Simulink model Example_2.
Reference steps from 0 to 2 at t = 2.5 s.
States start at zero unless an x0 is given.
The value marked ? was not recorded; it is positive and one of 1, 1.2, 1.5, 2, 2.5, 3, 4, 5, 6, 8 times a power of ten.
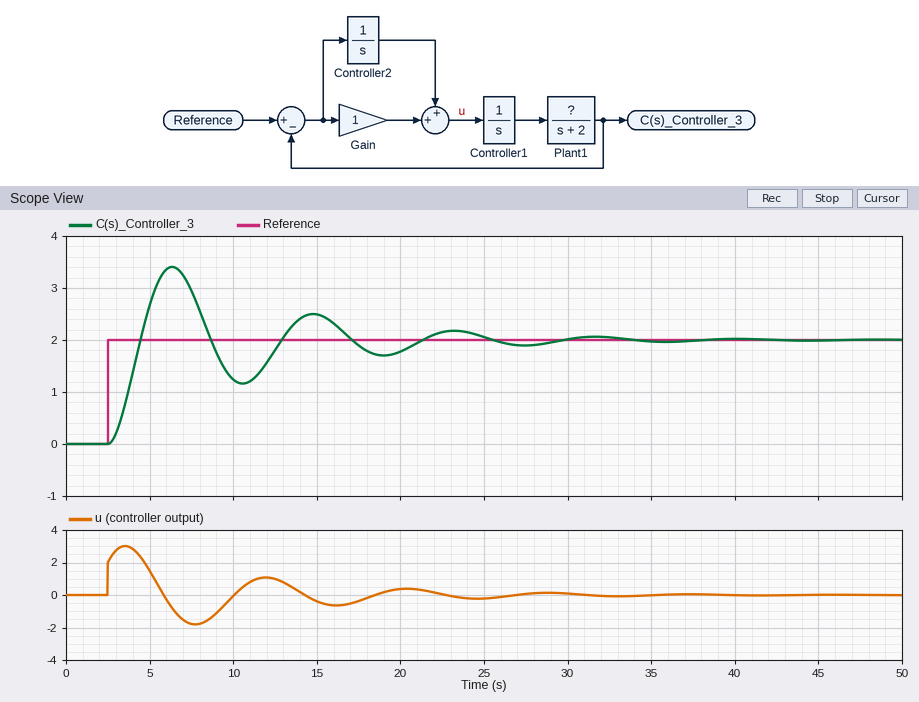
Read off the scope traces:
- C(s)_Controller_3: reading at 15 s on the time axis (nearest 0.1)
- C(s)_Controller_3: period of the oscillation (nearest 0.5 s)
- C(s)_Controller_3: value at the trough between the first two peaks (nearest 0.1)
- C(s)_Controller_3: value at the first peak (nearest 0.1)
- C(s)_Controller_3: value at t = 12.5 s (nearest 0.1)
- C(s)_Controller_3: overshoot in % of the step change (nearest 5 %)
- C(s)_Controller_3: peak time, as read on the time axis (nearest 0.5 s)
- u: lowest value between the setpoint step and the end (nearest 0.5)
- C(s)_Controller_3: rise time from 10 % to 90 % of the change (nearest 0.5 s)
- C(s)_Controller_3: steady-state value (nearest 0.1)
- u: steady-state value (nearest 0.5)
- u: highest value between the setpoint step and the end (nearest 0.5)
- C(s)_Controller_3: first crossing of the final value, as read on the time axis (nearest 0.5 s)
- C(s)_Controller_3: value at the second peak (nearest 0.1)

2.5
8.5 s
1.2
3.4
1.8
70 %
6.5 s
-2.0
1.5 s
2.0
0.0
3.0
4.5 s
2.5
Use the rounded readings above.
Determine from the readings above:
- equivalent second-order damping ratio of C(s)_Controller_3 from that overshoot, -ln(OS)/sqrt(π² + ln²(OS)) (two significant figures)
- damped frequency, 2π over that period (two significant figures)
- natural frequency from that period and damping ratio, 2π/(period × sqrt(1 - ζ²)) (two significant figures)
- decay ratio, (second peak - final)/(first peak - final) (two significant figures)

0.11
0.74 rad/s
0.74 rad/s
0.36
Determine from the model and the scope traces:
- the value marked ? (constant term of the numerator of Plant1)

1
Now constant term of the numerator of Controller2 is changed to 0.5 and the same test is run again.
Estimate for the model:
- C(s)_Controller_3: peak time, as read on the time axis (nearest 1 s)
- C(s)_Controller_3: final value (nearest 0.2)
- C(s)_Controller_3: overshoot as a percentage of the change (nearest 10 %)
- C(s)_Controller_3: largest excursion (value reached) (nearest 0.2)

7 s
2.0
50 %
3.0
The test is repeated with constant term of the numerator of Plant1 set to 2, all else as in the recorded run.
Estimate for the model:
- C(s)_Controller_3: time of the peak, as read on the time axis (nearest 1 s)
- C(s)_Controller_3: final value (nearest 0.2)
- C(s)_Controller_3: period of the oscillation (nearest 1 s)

5 s
2.0
6 s
